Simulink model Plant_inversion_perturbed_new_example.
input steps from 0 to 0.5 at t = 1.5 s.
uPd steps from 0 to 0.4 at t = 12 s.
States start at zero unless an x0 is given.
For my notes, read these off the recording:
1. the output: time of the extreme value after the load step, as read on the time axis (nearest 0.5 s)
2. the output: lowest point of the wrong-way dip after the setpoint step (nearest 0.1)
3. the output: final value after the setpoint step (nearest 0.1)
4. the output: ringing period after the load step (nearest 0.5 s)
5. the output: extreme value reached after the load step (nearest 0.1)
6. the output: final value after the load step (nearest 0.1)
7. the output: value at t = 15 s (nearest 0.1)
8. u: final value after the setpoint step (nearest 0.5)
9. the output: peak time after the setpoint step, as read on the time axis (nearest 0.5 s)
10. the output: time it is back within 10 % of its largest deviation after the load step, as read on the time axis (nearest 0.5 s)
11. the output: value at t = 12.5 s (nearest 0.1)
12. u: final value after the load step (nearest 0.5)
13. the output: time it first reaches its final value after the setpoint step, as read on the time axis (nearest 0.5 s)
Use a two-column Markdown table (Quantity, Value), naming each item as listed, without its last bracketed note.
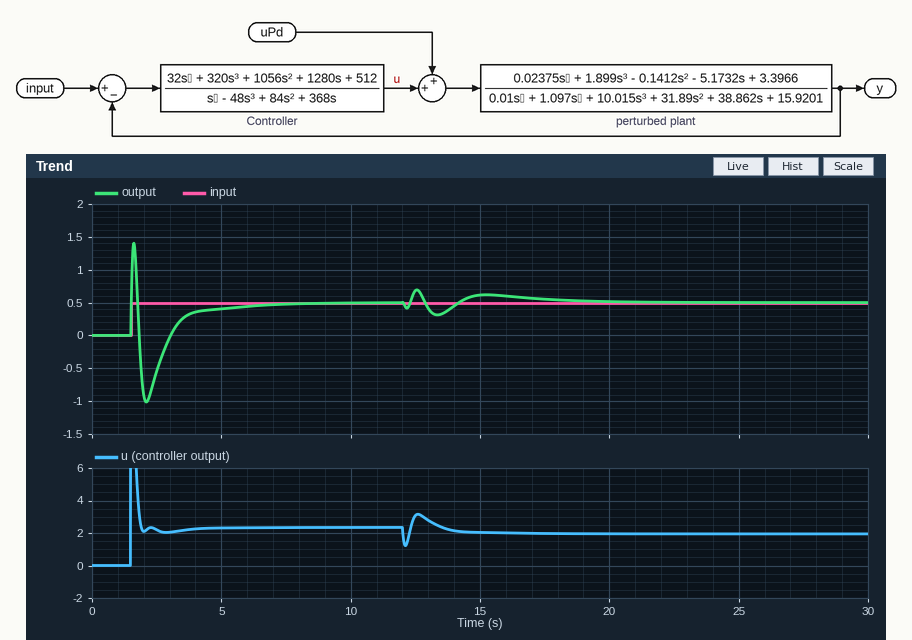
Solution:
| Quantity | Value |
|---|---|
| the output: time of the extreme value after the load step, as read on the time axis | 12.5 s |
| the output: lowest point of the wrong-way dip after the setpoint step | -1.0 |
| the output: final value after the setpoint step | 0.5 |
| the output: ringing period after the load step | 2.5 s |
| the output: extreme value reached after the load step | 0.7 |
| the output: final value after the load step | 0.5 |
| the output: value at t = 15 s | 0.6 |
| u: final value after the setpoint step | 2.5 |
| the output: peak time after the setpoint step, as read on the time axis | 1.5 s |
| the output: time it is back within 10 % of its largest deviation after the load step, as read on the time axis | 19.5 s |
| the output: value at t = 12.5 s | 0.7 |
| u: final value after the load step | 2.0 |
| the output: time it first reaches its final value after the setpoint step, as read on the time axis | 1.5 s |
